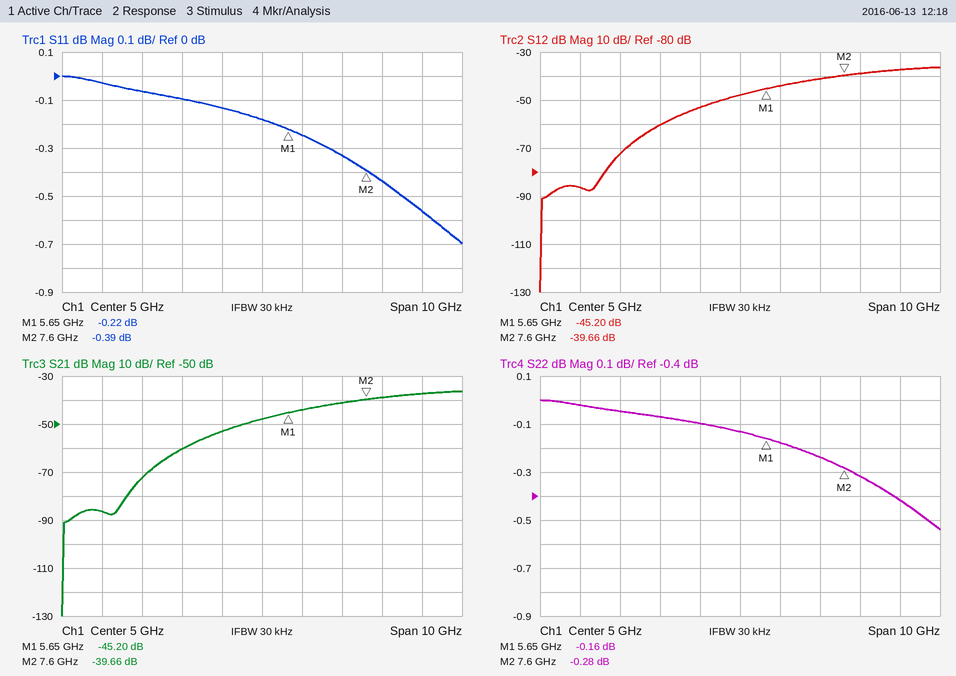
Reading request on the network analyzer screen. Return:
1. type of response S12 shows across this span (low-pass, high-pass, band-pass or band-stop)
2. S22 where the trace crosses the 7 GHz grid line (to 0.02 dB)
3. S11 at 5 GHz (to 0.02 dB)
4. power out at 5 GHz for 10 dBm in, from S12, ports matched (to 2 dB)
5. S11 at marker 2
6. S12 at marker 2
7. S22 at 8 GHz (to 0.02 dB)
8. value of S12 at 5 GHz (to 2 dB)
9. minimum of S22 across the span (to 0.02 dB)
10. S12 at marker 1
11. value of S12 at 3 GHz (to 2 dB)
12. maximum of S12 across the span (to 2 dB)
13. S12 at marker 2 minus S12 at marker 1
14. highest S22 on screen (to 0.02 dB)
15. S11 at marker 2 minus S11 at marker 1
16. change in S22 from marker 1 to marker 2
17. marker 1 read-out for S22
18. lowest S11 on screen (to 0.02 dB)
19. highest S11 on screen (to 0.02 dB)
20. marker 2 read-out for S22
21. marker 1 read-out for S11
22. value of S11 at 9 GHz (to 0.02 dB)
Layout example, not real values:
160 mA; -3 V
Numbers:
high-pass; -0.24 dB; -0.18 dB; -38 dBm; -0.39 dB; -39.66 dB; -0.32 dB; -48 dB; -0.54 dB; -45.20 dB; -60 dB; -36 dB; 5.54 dB; 0.00 dB; -0.17 dB; -0.12 dB; -0.16 dB; -0.70 dB; 0.00 dB; -0.28 dB; -0.22 dB; -0.56 dB
